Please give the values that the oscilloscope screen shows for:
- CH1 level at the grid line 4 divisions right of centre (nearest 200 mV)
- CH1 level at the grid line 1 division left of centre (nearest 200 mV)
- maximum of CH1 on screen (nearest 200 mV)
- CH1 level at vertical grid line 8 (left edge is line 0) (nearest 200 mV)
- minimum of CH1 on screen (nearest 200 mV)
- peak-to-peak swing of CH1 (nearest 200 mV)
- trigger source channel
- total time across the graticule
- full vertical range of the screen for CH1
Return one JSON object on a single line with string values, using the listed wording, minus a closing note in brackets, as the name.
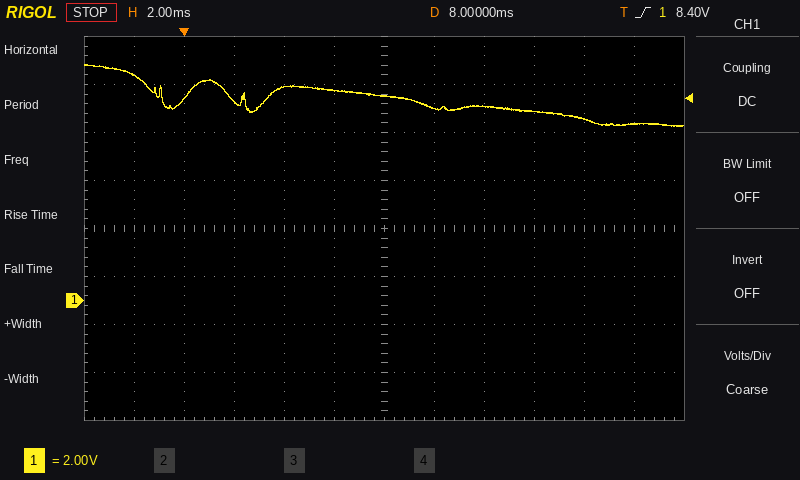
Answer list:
{"CH1 level at the grid line 4 divisions right of centre": "7.6 V", "CH1 level at the grid line 1 division left of centre": "8.8 V", "maximum of CH1 on screen": "9.8 V", "CH1 level at vertical grid line 8 (left edge is line 0)": "8.0 V", "minimum of CH1 on screen": "7.2 V", "peak-to-peak swing of CH1": "2.6 V", "trigger source channel": "CH1", "total time across the graticule": "24 ms", "full vertical range of the screen for CH1": "16 V"}
